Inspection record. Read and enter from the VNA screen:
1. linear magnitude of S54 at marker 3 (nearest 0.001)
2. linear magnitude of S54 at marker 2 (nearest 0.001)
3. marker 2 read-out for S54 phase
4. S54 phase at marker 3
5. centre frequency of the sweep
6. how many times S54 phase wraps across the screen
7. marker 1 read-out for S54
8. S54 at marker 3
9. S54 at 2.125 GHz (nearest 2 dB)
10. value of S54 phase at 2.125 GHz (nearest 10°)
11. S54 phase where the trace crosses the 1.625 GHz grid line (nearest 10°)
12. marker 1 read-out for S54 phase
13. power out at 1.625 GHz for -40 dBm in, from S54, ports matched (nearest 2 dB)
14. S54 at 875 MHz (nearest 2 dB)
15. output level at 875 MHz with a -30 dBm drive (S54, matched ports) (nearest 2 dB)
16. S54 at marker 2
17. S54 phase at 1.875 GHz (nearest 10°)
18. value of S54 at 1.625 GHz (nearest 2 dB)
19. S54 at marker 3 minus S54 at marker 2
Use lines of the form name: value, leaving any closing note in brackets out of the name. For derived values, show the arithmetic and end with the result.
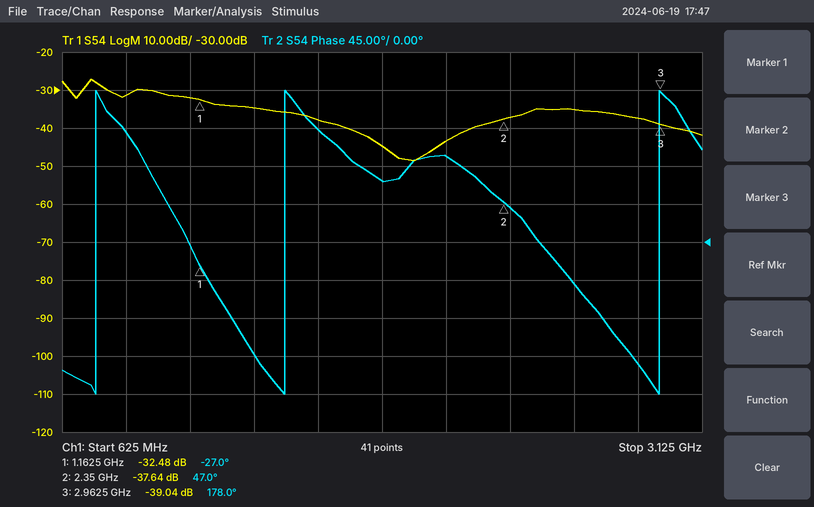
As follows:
linear magnitude of S54 at marker 3: 10^(-39.04/20) ≈ 0.011
linear magnitude of S54 at marker 2: 10^(-37.64/20) ≈ 0.013
marker 2 read-out for S54 phase: 47.0°
S54 phase at marker 3: 178.0°
centre frequency of the sweep: 1.875 GHz
how many times S54 phase wraps across the screen: 3
marker 1 read-out for S54: -32.48 dB
S54 at marker 3: -39.04 dB
S54 at 2.125 GHz: -44 dB
value of S54 phase at 2.125 GHz: 100°
S54 phase where the trace crosses the 1.625 GHz grid line: 130°
marker 1 read-out for S54 phase: -27.0°
power out at 1.625 GHz for -40 dBm in, from S54, ports matched: -40 dBm + (-38 dB) = -78 dBm
S54 at 875 MHz: -32 dB
output level at 875 MHz with a -30 dBm drive (S54, matched ports): -30 dBm + (-32 dB) = -62 dBm
S54 at marker 2: -37.64 dB
S54 phase at 1.875 GHz: 70°
value of S54 at 1.625 GHz: -38 dB
S54 at marker 3 minus S54 at marker 2: -39.04 − (-37.64) = -1.40 dB
